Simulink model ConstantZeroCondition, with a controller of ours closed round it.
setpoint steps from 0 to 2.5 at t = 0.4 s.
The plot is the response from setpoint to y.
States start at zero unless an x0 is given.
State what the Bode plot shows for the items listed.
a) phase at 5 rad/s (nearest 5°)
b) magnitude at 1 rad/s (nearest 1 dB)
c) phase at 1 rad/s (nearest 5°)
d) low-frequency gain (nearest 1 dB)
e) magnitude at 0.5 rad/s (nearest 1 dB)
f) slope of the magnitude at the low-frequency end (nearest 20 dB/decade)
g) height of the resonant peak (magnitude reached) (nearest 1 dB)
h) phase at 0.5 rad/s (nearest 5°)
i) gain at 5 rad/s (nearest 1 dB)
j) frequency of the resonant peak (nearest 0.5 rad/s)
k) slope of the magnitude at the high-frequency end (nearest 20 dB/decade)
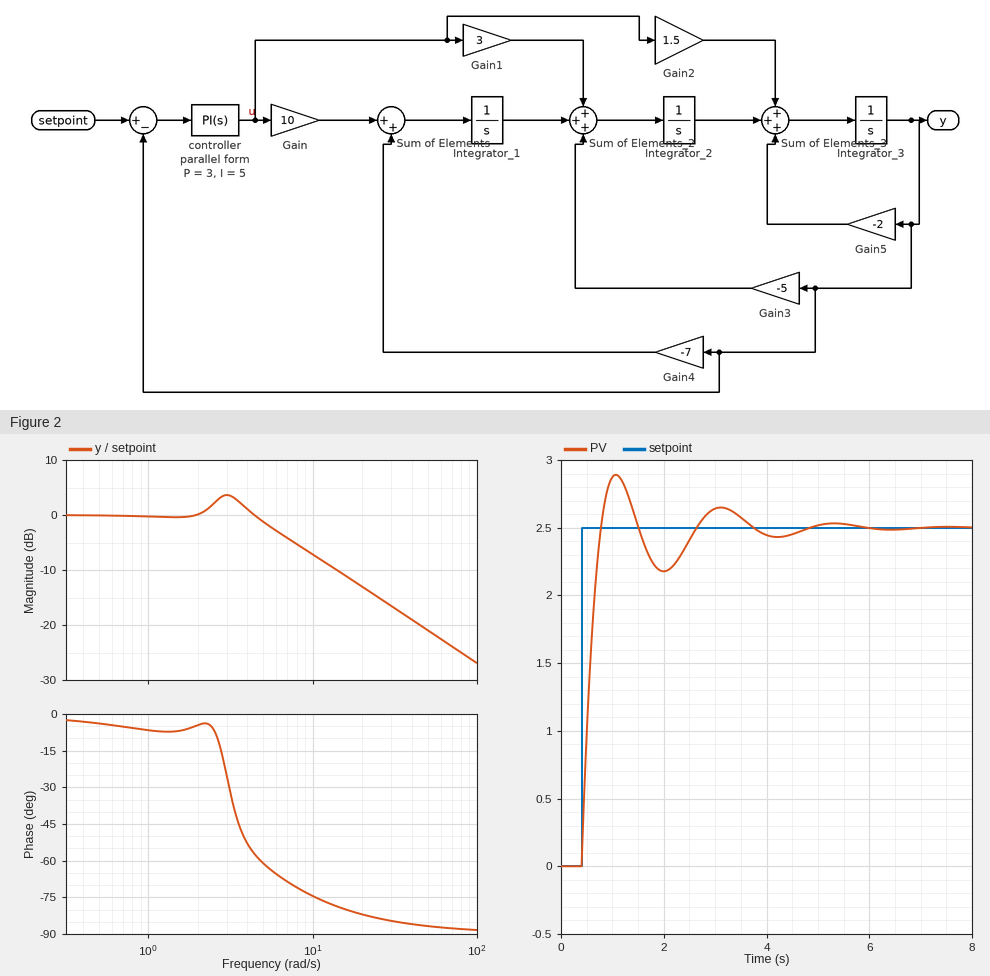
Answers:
-60°
0 dB
-5°
0 dB
0 dB
0 dB/decade
4 dB
-5°
-1 dB
3.0 rad/s
-20 dB/decade
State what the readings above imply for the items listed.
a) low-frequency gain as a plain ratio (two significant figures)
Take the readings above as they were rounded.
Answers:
1.0
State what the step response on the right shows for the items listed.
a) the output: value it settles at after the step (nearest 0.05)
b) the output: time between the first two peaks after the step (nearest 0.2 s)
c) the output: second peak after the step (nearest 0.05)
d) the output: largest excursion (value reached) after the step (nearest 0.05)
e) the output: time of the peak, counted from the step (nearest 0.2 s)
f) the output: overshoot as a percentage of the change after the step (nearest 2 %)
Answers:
2.50
2.0 s
2.65
2.90
0.6 s
16 %
